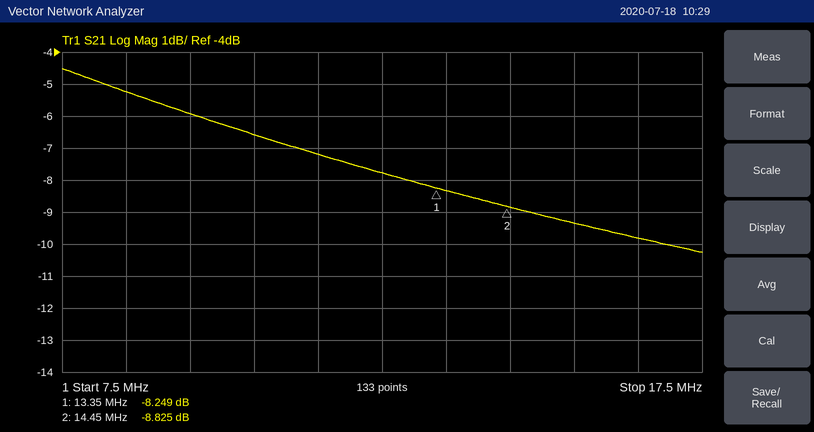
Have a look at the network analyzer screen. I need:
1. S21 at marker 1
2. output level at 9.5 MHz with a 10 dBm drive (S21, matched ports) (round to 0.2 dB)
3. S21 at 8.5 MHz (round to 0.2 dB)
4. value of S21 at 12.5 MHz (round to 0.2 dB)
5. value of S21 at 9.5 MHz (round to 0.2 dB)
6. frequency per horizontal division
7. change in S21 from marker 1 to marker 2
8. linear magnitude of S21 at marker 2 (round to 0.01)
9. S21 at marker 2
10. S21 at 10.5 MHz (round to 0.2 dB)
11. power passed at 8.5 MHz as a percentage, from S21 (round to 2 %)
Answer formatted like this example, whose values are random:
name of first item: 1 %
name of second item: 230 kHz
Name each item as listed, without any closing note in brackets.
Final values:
S21 at marker 1: -8.249 dB
output level at 9.5 MHz with a 10 dBm drive (S21, matched ports): 4.0 dBm
S21 at 8.5 MHz: -5.2 dB
value of S21 at 12.5 MHz: -7.8 dB
value of S21 at 9.5 MHz: -6.0 dB
frequency per horizontal division: 1 MHz
change in S21 from marker 1 to marker 2: -0.576 dB
linear magnitude of S21 at marker 2: 0.36
S21 at marker 2: -8.825 dB
S21 at 10.5 MHz: -6.6 dB
power passed at 8.5 MHz as a percentage, from S21: 30 %
